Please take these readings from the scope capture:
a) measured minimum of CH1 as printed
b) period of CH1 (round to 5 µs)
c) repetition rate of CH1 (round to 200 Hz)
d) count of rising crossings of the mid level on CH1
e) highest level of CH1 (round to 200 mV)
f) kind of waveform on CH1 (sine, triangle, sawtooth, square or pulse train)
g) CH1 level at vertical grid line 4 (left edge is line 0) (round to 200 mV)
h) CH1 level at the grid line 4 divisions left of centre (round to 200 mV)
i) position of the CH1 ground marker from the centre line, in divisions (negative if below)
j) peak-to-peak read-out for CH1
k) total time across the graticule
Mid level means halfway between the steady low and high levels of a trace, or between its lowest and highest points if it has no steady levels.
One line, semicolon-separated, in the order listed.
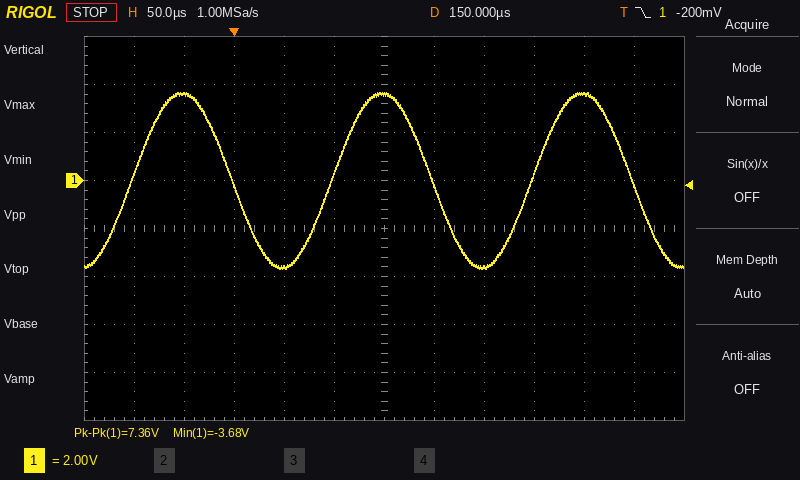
-3.68 V; 200 µs; 5.0 kHz; 3; 3.6 V; sine; -3.6 V; 3.6 V; +1.0 div; 7.36 V; 600 µs
